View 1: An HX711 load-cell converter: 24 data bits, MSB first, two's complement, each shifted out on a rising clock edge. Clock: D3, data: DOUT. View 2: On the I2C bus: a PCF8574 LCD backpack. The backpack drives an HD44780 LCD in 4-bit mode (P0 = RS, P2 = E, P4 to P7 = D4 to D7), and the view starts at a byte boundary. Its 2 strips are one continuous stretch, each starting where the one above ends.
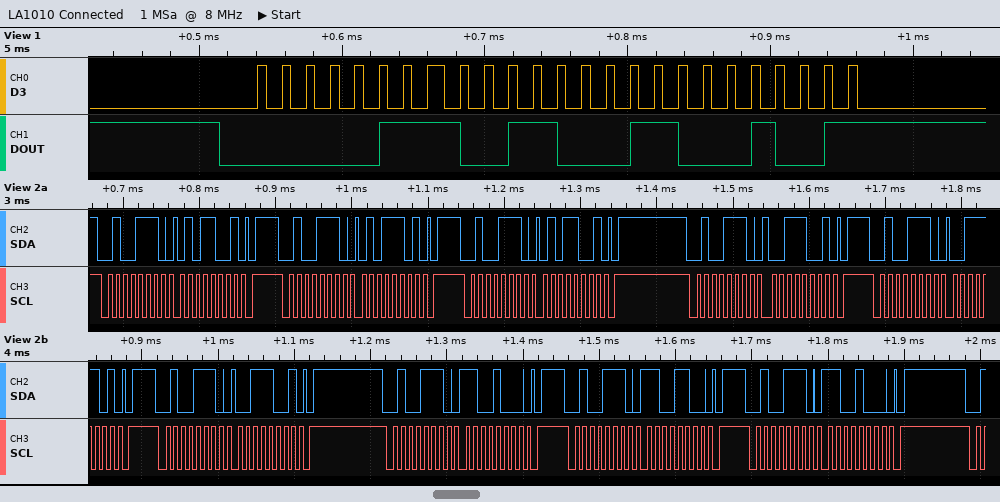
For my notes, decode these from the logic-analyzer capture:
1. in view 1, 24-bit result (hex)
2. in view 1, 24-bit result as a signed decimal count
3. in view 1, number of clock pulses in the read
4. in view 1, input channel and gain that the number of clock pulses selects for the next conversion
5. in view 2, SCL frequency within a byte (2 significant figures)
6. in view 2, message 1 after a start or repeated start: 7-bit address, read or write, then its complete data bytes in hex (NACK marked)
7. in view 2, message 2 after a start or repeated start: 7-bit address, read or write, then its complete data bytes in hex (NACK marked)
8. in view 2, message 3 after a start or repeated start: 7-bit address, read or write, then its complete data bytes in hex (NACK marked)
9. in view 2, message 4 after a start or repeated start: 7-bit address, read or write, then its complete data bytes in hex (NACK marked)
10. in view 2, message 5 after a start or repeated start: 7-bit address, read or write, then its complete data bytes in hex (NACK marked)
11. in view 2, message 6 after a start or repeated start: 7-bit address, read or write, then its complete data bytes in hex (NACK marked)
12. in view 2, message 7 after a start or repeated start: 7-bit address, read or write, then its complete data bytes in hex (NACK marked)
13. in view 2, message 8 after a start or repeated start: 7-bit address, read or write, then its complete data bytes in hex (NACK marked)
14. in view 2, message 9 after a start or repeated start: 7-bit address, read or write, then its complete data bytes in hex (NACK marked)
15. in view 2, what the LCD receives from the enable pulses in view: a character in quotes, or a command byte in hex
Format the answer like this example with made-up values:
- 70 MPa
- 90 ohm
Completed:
- 0x073189
- 471433
- 25
- channel A, gain 128
- 100 kHz
- 0x27 write: 59
- 0x27 write: 5D
- 0x27 write: 59
- 0x27 write: 39
- 0x27 write: 3D
- 0x27 write: 39
- 0x27 write: C8
- 0x27 write: CC
- 0x27 write: C8
- 'S'
